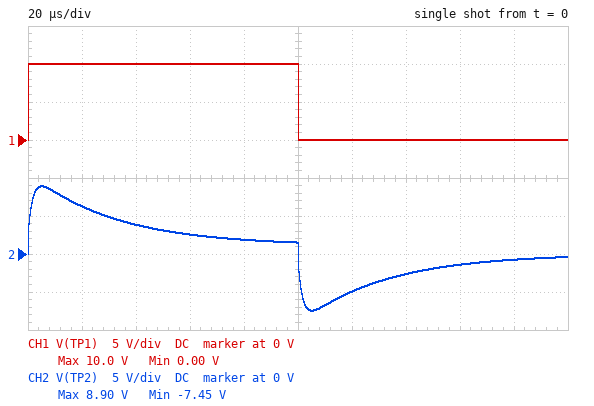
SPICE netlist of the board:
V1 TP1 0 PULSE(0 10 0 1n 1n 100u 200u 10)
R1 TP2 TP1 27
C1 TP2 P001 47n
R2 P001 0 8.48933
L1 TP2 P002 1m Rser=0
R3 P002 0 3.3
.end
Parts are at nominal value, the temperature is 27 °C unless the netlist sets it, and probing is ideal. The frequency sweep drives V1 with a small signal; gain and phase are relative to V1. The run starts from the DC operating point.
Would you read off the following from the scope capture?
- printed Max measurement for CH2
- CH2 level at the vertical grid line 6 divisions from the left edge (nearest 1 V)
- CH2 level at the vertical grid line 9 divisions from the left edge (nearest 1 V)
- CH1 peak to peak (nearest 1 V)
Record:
8.90 V
-5 V
-1 V
10 V
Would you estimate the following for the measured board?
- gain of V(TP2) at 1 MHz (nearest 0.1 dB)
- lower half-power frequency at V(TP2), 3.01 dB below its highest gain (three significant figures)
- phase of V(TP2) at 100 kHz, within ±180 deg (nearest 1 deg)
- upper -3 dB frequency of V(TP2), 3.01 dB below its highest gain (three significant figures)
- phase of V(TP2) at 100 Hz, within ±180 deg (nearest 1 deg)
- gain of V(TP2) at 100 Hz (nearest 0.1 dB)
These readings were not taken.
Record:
-11.8 dB
4.49 kHz
-31 deg
108 kHz
10 deg
-19.1 dB
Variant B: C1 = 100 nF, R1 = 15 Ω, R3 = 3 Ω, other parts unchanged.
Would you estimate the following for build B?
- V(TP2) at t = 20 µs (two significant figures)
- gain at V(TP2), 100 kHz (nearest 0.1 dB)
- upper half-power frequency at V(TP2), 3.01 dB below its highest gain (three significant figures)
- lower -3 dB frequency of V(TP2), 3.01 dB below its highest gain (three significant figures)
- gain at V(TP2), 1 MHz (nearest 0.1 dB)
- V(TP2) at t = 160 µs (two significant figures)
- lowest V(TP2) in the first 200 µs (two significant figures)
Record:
7.8 V
-3.9 dB
83.5 kHz
2.64 kHz
-8.7 dB
-2.5 V
-6.2 V
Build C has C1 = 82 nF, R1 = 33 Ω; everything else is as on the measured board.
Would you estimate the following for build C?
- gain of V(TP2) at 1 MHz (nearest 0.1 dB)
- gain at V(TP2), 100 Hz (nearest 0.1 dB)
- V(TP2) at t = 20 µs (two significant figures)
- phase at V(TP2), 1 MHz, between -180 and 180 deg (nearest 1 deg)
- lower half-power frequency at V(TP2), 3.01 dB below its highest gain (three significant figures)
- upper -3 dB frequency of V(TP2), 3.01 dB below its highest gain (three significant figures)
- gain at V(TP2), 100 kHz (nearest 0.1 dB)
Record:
-13.6 dB
-20.7 dB
6.1 V
-10 deg
5.04 kHz
55.7 kHz
-6.6 dB
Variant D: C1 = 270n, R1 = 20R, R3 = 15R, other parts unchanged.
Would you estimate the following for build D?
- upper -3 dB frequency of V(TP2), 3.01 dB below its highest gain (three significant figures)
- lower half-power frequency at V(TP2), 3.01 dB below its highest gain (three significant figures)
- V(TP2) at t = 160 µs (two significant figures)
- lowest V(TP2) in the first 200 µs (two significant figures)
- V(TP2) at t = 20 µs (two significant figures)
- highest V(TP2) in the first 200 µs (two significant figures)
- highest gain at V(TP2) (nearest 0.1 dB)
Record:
30.4 kHz
3.15 kHz
-880 mV
-3.5 V
7.7 V
7.8 V
-1.0 dB
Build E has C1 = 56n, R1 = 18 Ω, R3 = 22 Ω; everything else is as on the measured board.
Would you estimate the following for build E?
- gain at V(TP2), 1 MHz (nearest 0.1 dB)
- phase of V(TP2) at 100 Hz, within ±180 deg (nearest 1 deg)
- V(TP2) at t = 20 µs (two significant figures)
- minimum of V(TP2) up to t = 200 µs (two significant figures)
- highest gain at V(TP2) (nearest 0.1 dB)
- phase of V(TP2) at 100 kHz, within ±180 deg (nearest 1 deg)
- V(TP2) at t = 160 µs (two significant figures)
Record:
-9.5 dB
1 deg
7.7 V
-3.7 V
-0.2 dB
-25 deg
-420 mV
